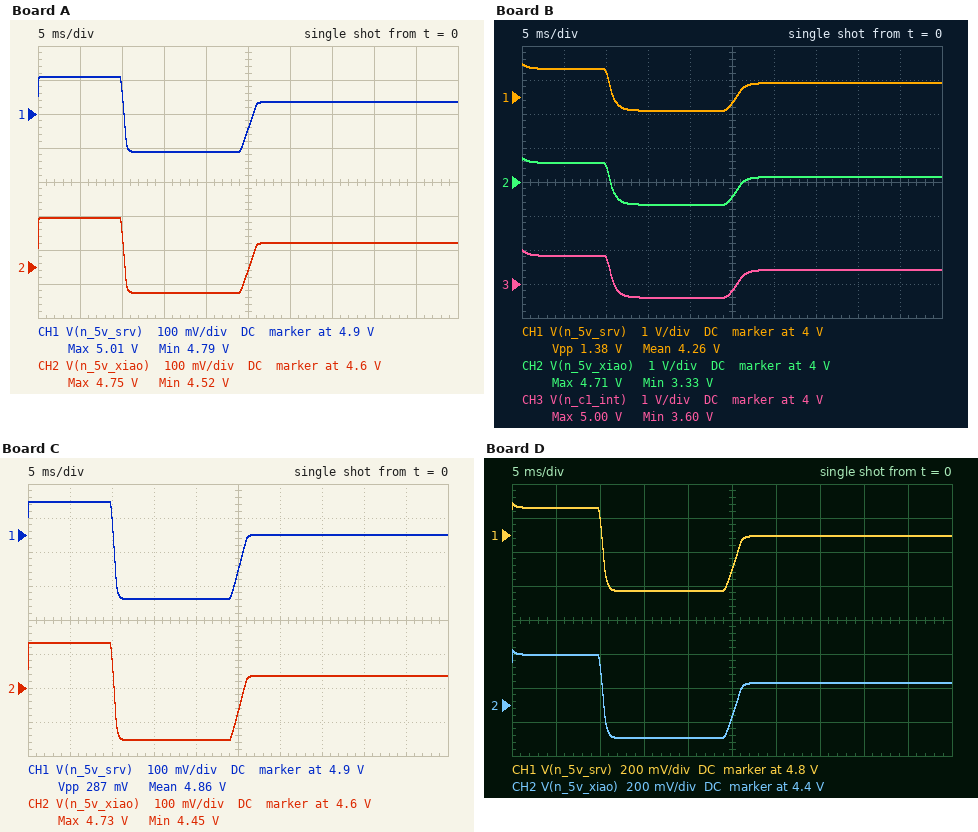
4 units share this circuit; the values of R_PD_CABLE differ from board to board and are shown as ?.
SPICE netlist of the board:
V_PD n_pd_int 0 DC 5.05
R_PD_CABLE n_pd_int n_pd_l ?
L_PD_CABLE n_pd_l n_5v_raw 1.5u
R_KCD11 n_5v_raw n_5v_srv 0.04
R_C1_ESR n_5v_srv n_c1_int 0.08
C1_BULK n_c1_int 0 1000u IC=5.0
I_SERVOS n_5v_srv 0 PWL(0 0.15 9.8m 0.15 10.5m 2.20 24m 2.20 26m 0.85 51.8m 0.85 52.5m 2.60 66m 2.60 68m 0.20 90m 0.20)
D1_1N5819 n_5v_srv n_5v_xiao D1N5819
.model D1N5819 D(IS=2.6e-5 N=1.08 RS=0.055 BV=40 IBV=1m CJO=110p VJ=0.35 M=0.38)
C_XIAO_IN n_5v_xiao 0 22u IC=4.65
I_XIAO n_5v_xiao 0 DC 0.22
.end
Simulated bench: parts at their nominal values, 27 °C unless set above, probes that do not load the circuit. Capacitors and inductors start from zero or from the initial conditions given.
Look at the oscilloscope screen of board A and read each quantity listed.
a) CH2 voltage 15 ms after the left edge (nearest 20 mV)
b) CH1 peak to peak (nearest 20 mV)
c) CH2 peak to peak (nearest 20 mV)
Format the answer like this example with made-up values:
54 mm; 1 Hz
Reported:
4.52 V; 220 mV; 220 mV
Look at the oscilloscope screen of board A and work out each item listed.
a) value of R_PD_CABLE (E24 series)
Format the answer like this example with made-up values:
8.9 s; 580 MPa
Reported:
0.068 Ω
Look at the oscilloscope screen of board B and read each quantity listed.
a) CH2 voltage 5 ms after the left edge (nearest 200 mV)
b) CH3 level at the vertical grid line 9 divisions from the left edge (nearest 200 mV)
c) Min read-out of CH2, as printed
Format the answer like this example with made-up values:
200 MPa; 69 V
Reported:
4.6 V; 4.4 V; 3.33 V
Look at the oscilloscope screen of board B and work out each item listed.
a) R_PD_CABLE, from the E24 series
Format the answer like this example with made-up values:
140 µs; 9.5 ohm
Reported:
0.56 Ω
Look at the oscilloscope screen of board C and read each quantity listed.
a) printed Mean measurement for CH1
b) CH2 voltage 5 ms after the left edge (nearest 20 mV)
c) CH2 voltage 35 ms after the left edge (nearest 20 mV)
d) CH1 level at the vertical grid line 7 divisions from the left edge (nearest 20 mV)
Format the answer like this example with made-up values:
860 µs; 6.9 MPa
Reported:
4.86 V; 4.74 V; 4.64 V; 4.90 V
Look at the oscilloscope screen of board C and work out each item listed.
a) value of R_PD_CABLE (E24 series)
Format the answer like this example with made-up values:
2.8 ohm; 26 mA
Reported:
0.1 Ω
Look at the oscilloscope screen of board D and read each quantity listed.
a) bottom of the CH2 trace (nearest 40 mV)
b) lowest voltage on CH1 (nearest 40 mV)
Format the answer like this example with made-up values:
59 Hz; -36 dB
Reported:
4.20 V; 4.48 V
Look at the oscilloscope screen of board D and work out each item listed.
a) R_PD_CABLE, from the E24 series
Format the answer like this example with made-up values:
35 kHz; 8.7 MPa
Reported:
0.2 Ω
